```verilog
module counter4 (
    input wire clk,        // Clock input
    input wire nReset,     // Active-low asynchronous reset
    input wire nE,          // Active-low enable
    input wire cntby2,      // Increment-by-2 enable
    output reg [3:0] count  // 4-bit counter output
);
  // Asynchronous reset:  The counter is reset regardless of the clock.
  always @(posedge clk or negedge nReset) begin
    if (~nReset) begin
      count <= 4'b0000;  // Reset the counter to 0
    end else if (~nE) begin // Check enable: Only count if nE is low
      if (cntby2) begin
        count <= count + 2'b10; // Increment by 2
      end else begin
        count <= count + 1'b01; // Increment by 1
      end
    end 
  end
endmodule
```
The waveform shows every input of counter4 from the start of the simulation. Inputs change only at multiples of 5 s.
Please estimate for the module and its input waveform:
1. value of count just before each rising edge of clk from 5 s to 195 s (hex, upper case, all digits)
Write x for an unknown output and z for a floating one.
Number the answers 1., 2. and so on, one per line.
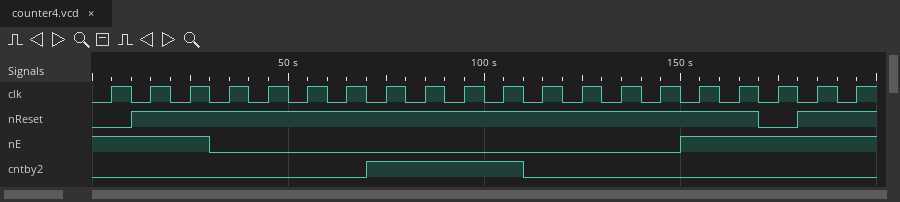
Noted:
1. 0, 0, 0, 0, 1, 2, 3, 4, 6, 8, A, C, D, E, F, 0, 0, 0, 0, 0
